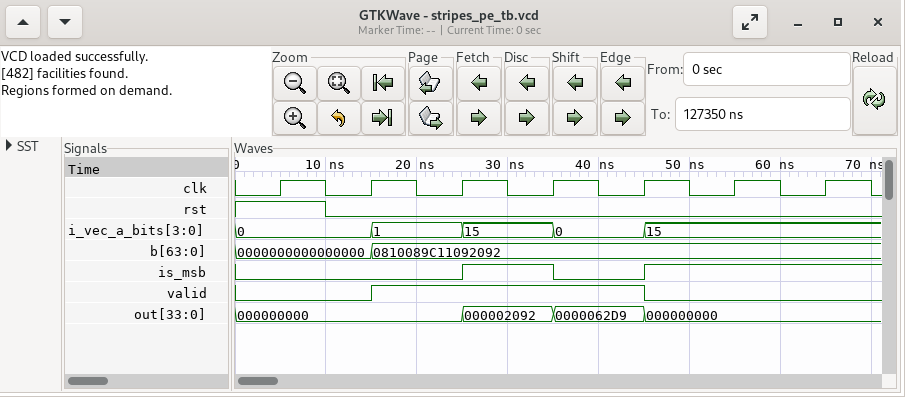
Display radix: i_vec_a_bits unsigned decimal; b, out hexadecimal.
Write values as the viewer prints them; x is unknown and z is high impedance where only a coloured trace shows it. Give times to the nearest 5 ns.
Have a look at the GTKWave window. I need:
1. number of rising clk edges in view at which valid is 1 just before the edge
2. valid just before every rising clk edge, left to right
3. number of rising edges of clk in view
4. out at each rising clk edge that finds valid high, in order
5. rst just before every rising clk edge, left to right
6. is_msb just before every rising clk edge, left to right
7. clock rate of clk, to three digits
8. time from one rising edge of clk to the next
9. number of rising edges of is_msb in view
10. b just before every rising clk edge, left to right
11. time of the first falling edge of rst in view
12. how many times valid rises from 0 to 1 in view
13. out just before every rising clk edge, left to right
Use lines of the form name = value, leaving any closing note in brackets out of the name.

number of rising clk edges in view at which valid is 1 just before the edge = 3
valid just before every rising clk edge, left to right = 0 0 1 1 1 0 0
number of rising edges of clk in view = 7
out at each rising clk edge that finds valid high, in order = 000000000, 000002092, 0000062D9
rst just before every rising clk edge, left to right = 1 0 0 0 0 0 0
is_msb just before every rising clk edge, left to right = 0 0 0 1 0 1 1
clock rate of clk, to three digits = 100 MHz
time from one rising edge of clk to the next = 10 ns
number of rising edges of is_msb in view = 2
b just before every rising clk edge, left to right = 0000000000000000, 0000000000000000, 0810089C11092092, 0810089C11092092, 0810089C11092092, 0810089C11092092, 0810089C11092092
time of the first falling edge of rst in view = 10 ns
how many times valid rises from 0 to 1 in view = 1
out just before every rising clk edge, left to right = 000000000, 000000000, 000000000, 000002092, 0000062D9, 000000000, 000000000
